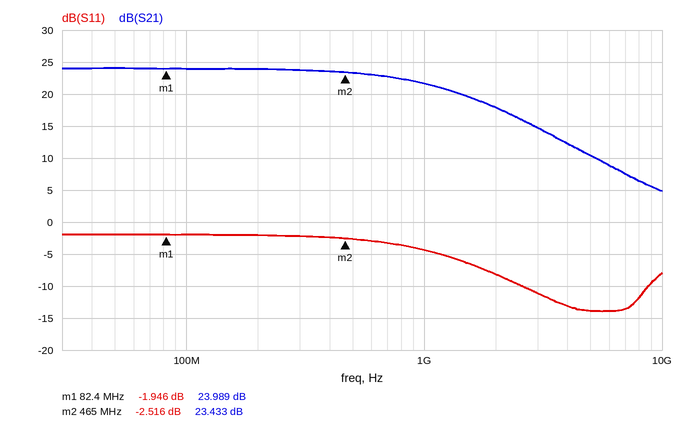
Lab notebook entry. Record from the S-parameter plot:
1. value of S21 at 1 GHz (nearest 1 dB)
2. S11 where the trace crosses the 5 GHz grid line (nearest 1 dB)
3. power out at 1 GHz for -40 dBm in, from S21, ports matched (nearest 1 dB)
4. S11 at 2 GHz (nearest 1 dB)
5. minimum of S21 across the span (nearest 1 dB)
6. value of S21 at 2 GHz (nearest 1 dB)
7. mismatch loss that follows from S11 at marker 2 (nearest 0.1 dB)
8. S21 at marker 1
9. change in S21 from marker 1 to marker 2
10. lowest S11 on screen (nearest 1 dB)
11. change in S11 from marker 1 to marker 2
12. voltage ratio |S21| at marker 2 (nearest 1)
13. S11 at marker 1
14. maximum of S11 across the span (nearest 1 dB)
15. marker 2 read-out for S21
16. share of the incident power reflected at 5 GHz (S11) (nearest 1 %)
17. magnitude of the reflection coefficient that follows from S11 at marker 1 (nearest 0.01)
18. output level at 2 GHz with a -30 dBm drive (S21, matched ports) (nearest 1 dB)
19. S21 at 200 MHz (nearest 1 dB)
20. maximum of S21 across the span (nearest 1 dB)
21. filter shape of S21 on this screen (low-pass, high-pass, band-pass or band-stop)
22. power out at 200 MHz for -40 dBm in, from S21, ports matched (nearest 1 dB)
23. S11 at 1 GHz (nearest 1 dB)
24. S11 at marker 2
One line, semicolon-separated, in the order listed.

22 dB; -14 dB; -18 dBm; -8 dB; 5 dB; 18 dB; 3.6 dB; 23.989 dB; -0.556 dB; -14 dB; -0.570 dB; 15; -1.946 dB; -2 dB; 23.433 dB; 4 %; 0.80; -12 dBm; 24 dB; 24 dB; low-pass; -16 dBm; -4 dB; -2.516 dB
